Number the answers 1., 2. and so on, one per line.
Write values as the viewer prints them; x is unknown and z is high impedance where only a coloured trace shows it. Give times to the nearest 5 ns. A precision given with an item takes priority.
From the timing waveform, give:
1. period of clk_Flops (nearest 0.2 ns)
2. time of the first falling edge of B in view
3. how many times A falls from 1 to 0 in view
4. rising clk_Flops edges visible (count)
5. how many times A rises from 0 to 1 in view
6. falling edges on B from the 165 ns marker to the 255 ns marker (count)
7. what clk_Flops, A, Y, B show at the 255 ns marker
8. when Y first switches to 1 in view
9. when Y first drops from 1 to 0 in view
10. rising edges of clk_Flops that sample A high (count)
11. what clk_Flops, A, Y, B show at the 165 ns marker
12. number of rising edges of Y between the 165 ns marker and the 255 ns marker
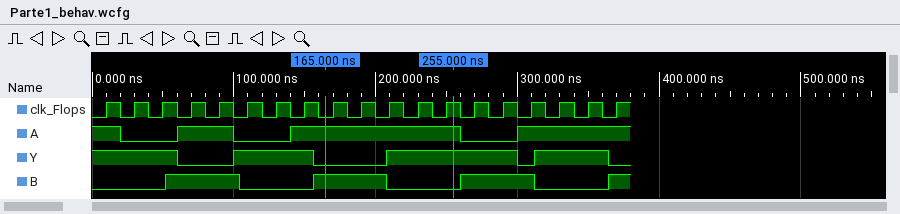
1. 20 ns
2. 105 ns
3. 3
4. 19
5. 3
6. 1
7. clk_Flops=1, A=1, Y=1, B=0
8. 100 ns
9. 60 ns
10. 13
11. clk_Flops=0, A=1, Y=0, B=1
12. 1
